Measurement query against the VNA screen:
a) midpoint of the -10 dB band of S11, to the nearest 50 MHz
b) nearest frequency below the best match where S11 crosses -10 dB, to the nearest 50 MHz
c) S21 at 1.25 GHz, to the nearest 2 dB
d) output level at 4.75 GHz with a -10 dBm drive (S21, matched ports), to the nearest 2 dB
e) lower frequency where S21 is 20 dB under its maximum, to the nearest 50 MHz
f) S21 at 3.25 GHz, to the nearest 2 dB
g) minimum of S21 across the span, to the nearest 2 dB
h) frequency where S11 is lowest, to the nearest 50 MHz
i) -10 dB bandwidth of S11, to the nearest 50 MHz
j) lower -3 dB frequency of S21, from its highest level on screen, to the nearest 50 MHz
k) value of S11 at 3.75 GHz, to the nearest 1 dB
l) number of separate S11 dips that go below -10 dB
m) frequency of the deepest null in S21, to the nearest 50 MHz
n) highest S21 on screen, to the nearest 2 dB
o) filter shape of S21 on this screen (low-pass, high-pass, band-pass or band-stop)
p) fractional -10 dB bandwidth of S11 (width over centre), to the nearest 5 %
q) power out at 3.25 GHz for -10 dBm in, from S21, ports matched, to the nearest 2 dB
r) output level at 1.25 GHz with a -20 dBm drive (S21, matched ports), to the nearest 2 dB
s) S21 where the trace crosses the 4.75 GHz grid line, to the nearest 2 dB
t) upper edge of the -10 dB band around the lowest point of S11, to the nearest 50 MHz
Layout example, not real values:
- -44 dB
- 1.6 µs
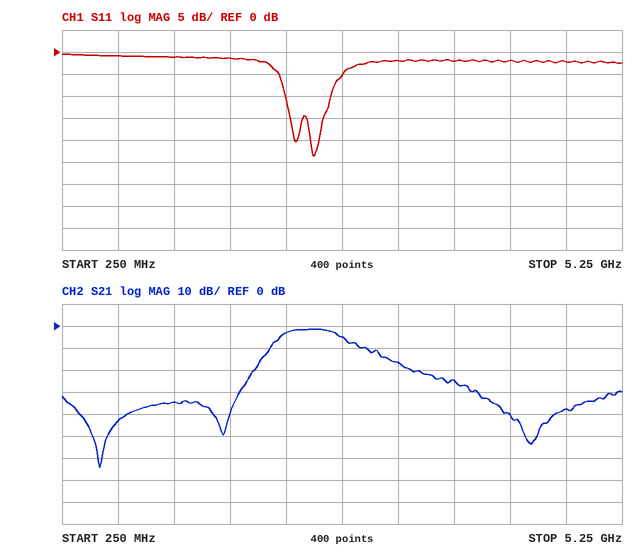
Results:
- 2.45 GHz
- 2.25 GHz
- -34 dB
- -48 dBm
- 1.95 GHz
- -16 dB
- -64 dB
- 2.50 GHz
- 400 MHz
- 2.20 GHz
- -2 dB
- 2
- 600 MHz
- -2 dB
- band-pass
- 15 %
- -26 dBm
- -54 dBm
- -38 dB
- 2.65 GHz
